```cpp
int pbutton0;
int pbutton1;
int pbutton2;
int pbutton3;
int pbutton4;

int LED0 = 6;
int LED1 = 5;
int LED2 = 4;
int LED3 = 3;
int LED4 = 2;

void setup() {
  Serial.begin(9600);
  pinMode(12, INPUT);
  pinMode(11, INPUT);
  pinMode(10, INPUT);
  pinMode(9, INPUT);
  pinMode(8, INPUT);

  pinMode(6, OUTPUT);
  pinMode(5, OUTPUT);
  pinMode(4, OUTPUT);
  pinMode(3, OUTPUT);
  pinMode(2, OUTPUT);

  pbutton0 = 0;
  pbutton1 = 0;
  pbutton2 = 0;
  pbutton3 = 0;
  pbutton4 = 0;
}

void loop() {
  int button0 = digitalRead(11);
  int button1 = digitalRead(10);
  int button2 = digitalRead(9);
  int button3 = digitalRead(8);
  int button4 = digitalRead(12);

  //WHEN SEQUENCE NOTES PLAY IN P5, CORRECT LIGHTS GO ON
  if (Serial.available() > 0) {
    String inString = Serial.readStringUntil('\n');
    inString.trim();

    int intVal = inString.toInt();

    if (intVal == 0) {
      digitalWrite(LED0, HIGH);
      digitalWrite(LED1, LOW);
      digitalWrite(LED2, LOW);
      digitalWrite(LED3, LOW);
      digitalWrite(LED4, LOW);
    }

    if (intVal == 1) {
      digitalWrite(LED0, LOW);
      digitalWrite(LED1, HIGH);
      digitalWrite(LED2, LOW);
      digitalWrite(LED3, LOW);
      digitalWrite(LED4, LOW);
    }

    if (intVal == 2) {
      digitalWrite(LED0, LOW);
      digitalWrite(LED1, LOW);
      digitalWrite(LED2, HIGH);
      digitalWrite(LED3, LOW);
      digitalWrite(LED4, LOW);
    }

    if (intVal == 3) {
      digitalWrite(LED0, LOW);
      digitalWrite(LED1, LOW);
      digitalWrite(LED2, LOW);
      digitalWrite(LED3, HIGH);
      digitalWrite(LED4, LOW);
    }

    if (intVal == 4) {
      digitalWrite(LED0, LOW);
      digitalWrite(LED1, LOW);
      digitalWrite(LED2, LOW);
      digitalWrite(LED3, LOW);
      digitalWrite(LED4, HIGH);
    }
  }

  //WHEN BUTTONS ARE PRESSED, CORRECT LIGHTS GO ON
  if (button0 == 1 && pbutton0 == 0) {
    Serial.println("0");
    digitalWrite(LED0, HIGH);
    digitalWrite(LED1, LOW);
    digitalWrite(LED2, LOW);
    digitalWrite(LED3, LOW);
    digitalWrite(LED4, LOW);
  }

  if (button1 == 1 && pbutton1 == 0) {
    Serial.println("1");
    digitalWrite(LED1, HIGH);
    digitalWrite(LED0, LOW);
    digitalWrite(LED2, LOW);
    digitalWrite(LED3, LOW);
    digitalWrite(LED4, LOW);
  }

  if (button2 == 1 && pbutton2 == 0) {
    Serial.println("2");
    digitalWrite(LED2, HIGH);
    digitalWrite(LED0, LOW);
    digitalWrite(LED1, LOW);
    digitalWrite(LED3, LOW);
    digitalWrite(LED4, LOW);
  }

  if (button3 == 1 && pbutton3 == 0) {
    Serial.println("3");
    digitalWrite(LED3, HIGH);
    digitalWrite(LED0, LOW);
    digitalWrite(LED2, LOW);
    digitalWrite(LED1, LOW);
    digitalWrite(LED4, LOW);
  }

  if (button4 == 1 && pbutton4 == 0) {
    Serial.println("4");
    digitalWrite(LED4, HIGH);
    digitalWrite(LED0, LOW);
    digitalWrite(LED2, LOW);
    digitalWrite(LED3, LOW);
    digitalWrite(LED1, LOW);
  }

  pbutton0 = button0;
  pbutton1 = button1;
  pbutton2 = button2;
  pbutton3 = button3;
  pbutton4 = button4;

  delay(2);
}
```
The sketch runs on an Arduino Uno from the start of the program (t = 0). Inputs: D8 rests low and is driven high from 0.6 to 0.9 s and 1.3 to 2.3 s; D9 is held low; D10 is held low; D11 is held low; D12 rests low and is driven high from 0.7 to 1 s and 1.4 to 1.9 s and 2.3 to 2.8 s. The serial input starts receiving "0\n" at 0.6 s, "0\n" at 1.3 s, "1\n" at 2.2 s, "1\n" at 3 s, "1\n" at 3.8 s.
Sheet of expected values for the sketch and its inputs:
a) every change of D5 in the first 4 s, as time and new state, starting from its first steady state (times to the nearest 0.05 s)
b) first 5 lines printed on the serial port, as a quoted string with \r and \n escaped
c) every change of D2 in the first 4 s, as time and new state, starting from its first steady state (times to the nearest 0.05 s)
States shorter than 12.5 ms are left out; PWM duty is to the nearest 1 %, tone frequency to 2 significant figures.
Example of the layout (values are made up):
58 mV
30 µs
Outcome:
0 s low; 2.2 s high; 2.3 s low; 3 s high
"3\r\n4\r\n3\r\n4\r\n4\r\n"
0 s low; 0.7 s high; 1.3 s low; 1.4 s high; 2.2 s low; 2.3 s high; 3 s low
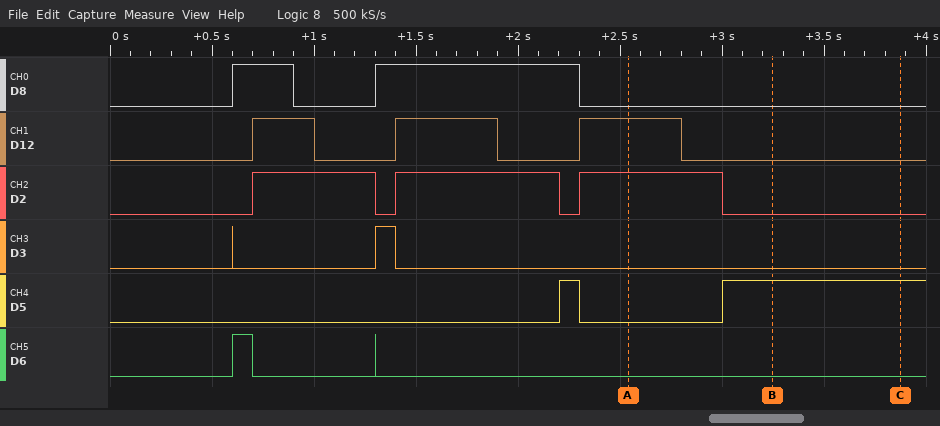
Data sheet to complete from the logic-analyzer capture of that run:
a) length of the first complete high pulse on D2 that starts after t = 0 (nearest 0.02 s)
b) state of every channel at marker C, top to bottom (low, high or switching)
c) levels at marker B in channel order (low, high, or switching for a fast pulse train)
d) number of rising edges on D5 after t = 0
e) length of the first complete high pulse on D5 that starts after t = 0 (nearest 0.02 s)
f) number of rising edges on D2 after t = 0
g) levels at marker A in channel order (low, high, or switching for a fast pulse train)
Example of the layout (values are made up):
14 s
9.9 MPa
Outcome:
0.60 s
D8 low, D12 low, D2 low, D3 low, D5 high, D6 low
D8 low, D12 low, D2 low, D3 low, D5 high, D6 low
2
0.10 s
3
D8 low, D12 high, D2 high, D3 low, D5 low, D6 low
